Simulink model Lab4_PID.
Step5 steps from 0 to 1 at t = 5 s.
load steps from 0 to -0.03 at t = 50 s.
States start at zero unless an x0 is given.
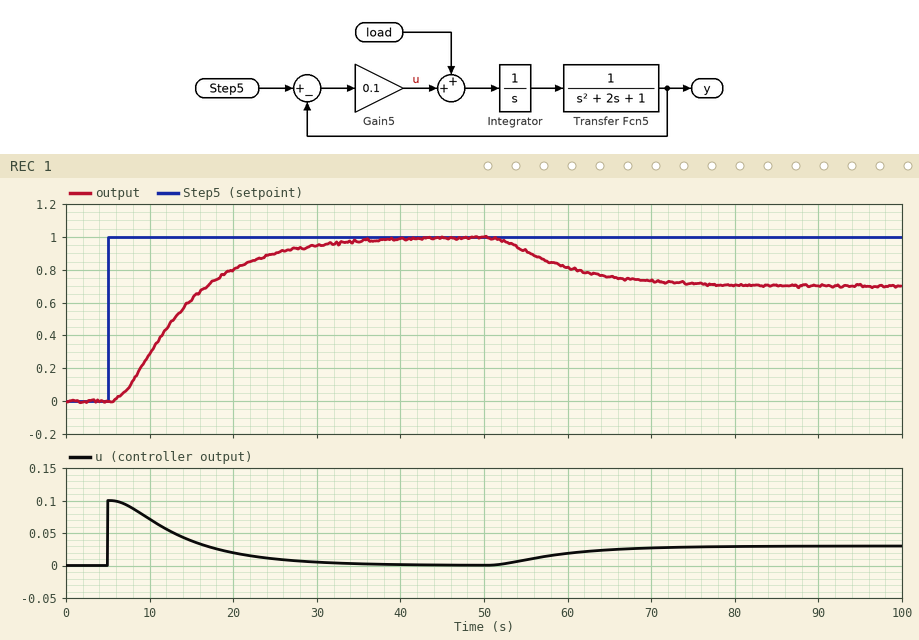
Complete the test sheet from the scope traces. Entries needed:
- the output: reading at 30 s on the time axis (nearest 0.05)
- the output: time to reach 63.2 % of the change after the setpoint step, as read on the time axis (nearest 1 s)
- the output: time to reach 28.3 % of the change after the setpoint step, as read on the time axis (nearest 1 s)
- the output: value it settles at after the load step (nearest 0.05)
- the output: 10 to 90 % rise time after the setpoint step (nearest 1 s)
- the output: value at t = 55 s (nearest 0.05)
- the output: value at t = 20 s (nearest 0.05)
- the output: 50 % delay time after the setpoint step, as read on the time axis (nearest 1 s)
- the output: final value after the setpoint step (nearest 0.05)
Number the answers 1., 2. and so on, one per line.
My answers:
1. 0.95
2. 15 s
3. 10 s
4. 0.70
5. 17 s
6. 0.90
7. 0.80
8. 13 s
9. 1.00
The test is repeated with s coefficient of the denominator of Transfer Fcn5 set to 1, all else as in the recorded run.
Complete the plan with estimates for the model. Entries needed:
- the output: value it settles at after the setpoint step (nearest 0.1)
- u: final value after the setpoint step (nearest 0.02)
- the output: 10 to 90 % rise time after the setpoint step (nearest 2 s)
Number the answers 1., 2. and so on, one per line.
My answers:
1. 1.0
2. 0.00
3. 20 s
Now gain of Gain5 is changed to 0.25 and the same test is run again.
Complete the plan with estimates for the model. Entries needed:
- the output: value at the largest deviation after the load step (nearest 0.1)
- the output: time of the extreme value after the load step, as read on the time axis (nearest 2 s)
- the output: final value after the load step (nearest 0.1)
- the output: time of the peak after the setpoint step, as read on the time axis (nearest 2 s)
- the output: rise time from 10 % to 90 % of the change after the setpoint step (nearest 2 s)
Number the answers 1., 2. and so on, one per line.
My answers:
1. 0.9
2. 62 s
3. 0.9
4. 16 s
5. 6 s
